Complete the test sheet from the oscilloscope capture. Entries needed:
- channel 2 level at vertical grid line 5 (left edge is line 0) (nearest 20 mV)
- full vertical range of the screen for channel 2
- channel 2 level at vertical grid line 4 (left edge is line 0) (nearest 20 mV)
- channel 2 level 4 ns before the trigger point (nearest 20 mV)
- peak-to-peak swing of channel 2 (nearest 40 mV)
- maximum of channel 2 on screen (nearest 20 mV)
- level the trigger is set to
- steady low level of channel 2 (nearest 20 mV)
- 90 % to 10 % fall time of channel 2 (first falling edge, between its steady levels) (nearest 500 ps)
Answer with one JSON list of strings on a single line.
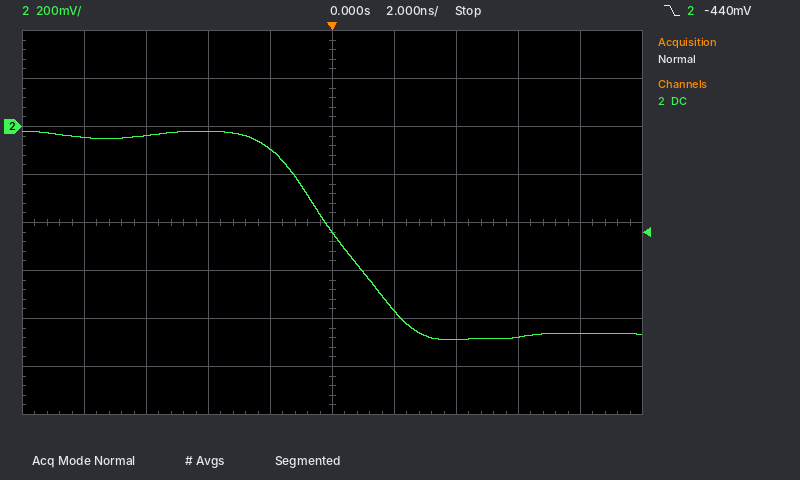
["-440 mV", "1.6 V", "-100 mV", "-20 mV", "880 mV", "-20 mV", "-440 mV", "-860 mV", "4.0 ns"]
